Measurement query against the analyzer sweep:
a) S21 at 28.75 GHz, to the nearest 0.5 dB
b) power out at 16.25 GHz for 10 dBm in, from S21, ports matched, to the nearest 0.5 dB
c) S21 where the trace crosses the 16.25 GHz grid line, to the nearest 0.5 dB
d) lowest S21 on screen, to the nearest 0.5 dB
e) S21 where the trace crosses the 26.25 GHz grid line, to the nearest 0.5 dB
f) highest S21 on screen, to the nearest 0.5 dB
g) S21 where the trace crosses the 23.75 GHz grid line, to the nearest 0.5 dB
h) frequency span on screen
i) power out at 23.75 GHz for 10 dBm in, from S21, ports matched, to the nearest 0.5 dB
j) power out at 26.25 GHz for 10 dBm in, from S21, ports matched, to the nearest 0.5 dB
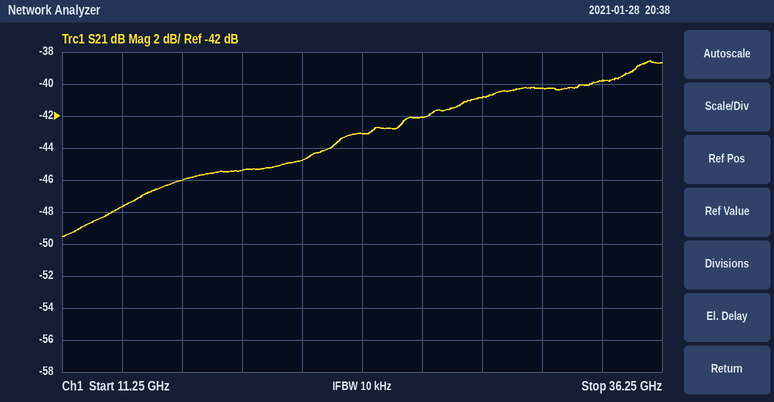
-41.0 dB
-36.0 dBm
-46.0 dB
-49.5 dB
-42.0 dB
-38.5 dB
-43.0 dB
25 GHz
-33.0 dBm
-32.0 dBm
